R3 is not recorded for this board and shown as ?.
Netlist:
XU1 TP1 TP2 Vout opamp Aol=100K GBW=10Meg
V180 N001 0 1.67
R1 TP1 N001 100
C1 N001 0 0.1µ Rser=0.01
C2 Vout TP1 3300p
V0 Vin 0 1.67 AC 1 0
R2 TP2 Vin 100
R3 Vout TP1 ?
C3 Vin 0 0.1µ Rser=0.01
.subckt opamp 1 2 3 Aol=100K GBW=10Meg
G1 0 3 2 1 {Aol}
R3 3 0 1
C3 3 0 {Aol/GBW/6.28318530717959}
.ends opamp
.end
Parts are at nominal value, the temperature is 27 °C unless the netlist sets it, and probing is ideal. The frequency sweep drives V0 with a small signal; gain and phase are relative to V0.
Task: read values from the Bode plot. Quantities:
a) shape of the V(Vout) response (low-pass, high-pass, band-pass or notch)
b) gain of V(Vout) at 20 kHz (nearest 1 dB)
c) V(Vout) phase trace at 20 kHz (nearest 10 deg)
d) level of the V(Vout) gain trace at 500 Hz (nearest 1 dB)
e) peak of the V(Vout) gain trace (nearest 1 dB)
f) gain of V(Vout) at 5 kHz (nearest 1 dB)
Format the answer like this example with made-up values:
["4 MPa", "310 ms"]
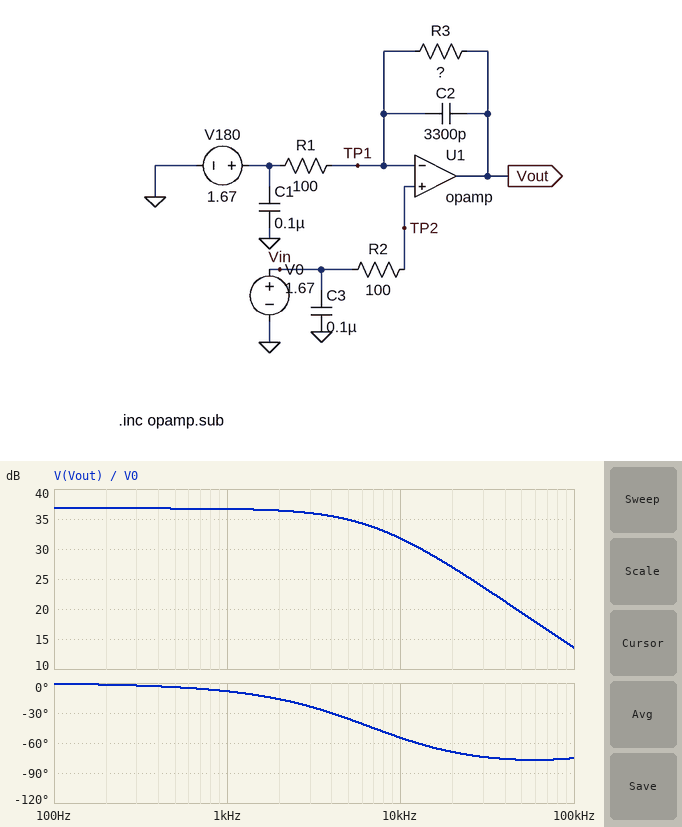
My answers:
["low-pass", "27 dB", "-70 deg", "37 dB", "37 dB", "35 dB"]
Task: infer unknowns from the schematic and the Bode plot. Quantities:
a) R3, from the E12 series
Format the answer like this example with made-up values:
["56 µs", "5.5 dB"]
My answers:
["6.8 kΩ"]
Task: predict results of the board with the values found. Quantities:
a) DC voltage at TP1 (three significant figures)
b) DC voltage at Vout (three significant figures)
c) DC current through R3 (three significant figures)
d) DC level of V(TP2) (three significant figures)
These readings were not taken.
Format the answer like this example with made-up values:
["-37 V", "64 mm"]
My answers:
["1.67 V", "1.67 V", "167 nA", "1.67 V"]
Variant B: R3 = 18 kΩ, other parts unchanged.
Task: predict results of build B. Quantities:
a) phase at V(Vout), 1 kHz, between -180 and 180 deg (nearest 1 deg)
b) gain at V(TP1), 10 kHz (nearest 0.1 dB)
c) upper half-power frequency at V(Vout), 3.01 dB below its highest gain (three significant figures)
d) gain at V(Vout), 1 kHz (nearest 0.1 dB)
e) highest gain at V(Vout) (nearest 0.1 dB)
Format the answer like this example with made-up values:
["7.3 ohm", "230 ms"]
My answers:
["-21 deg", "-0.4 dB", "2.56 kHz", "44.5 dB", "45.1 dB"]
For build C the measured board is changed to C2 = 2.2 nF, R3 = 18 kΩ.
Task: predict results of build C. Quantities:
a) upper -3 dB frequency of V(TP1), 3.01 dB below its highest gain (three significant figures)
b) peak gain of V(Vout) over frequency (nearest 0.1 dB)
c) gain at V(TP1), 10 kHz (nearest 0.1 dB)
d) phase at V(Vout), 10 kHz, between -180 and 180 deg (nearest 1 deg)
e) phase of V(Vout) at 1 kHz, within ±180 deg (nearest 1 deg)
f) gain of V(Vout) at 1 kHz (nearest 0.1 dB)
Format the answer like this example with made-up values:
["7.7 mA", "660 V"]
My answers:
["9.26 MHz", "45.1 dB", "-0.5 dB", "-69 deg", "-15 deg", "44.8 dB"]
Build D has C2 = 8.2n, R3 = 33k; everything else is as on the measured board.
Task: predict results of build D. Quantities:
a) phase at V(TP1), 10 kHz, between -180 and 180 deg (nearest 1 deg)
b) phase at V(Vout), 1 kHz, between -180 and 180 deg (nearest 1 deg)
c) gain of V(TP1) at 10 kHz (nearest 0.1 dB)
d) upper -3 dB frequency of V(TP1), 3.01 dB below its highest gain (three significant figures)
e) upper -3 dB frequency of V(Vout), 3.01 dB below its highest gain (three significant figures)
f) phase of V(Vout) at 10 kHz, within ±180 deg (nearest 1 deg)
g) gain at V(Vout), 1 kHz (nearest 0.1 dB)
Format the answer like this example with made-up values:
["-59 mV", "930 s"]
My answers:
["0 deg", "-60 deg", "-0.2 dB", "9.87 MHz", "579 Hz", "-84 deg", "44.4 dB"]
